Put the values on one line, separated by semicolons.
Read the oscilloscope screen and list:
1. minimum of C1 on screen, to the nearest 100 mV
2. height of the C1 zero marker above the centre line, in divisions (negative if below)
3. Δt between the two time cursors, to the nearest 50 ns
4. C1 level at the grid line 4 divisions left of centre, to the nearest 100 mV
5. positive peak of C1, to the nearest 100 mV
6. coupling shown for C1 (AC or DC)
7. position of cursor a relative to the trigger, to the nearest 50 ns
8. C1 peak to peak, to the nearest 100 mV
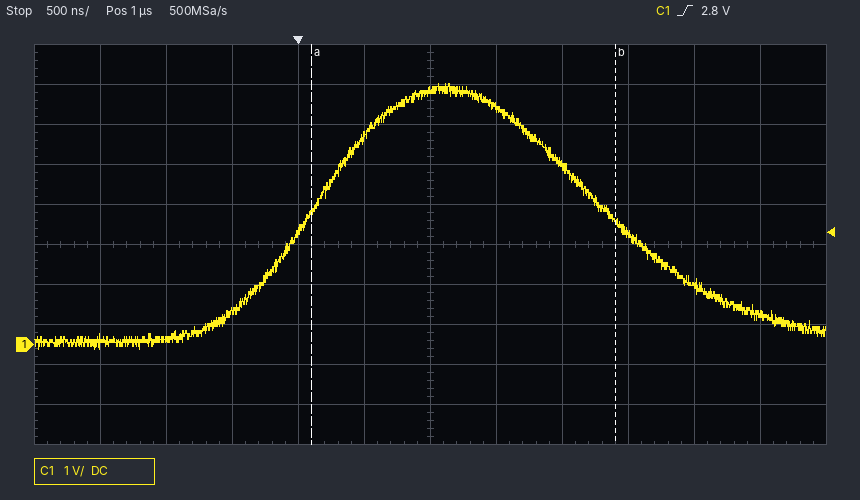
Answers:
-100 mV; -2.5 div; 2.30 µs; 100 mV; 6.5 V; DC; +100 ns; 6.6 V
